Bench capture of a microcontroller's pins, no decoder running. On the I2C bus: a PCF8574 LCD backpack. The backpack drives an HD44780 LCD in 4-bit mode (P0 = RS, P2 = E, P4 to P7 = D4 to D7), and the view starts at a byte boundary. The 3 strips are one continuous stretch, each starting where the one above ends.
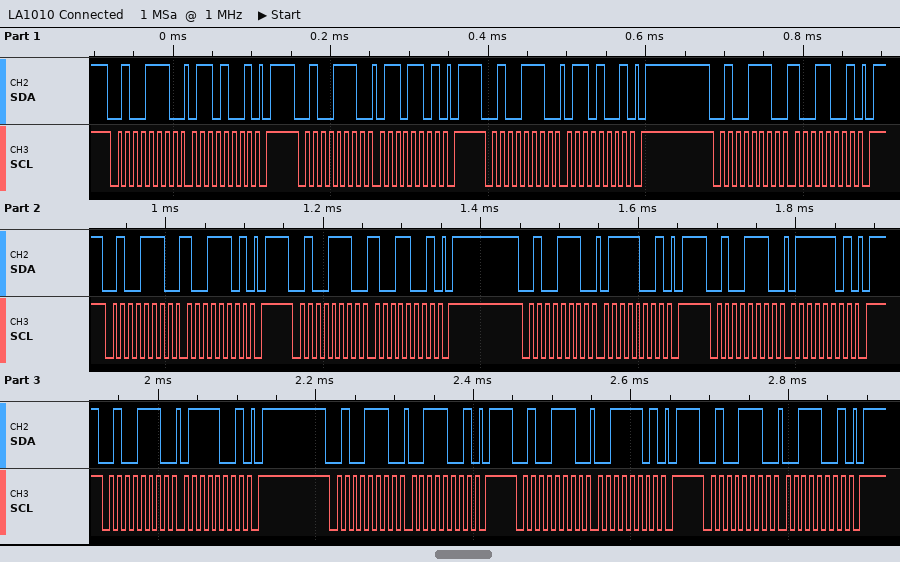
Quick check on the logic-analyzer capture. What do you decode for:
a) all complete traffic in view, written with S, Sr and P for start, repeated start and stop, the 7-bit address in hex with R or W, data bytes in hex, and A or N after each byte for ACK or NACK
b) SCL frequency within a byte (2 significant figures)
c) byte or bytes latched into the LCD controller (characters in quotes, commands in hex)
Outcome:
S 27W A 69 A P S 27W A 6D A P S 27W A 69 A P S 27W A 99 A P S 27W A 9D A P S 27W A 99 A P S 27W A 79 A P S 27W A 7D A P S 27W A 79 A P S 27W A 39 A P S 27W A 3D A P S 27W A 39 A P
100 kHz
'i' 's'
